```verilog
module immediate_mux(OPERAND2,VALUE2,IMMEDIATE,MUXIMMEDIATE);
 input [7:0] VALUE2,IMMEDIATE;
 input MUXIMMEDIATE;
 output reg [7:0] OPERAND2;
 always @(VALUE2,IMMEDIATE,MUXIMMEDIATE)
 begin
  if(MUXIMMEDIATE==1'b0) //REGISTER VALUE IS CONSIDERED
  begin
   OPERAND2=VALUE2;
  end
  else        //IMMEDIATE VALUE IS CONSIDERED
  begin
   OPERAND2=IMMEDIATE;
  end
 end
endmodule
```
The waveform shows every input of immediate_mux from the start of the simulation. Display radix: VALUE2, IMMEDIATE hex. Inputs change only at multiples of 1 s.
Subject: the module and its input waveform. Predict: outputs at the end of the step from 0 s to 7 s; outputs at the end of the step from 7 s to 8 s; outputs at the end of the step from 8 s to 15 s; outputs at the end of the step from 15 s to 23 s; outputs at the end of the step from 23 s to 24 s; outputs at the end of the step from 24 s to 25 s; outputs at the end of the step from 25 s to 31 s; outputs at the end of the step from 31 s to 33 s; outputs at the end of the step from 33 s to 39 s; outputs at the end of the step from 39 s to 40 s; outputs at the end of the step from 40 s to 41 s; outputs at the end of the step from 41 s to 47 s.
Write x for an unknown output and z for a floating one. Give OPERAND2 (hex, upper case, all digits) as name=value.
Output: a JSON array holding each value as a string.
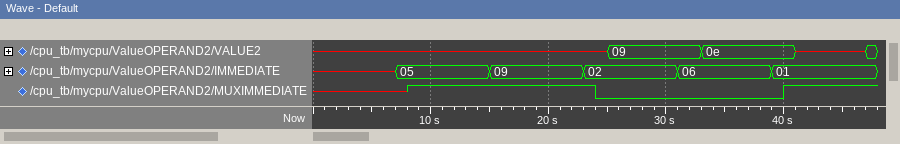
["OPERAND2=x", "OPERAND2=05", "OPERAND2=05", "OPERAND2=09", "OPERAND2=02", "OPERAND2=x", "OPERAND2=09", "OPERAND2=09", "OPERAND2=0E", "OPERAND2=0E", "OPERAND2=01", "OPERAND2=01"]
